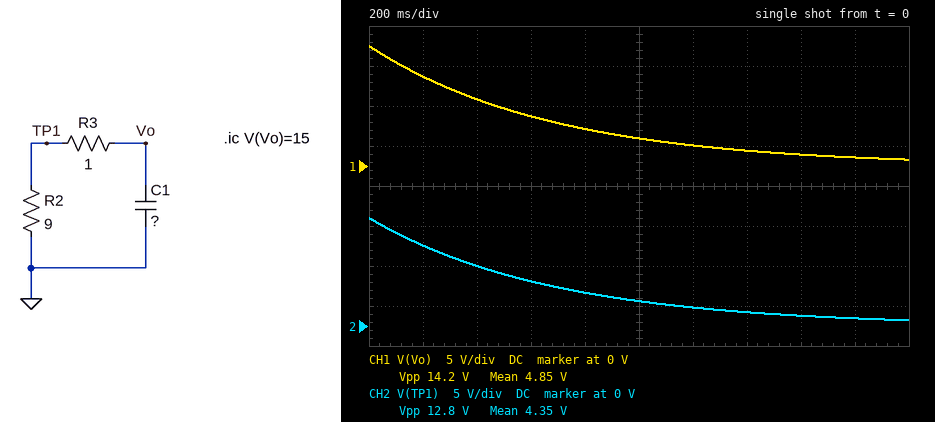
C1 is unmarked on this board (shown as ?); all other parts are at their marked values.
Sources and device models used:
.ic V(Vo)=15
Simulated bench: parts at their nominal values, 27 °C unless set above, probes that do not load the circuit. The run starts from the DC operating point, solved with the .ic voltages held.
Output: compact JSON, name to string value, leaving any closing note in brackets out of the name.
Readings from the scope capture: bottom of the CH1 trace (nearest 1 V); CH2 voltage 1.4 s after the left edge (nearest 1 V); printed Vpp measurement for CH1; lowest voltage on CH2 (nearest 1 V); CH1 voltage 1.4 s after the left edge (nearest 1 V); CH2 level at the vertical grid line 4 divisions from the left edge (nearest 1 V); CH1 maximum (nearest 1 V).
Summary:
{"bottom of the CH1 trace": "1 V", "CH2 voltage 1.4 s after the left edge": "2 V", "printed Vpp measurement for CH1": "14.2 V", "lowest voltage on CH2": "1 V", "CH1 voltage 1.4 s after the left edge": "2 V", "CH2 level at the vertical grid line 4 divisions from the left edge": "4 V", "CH1 maximum": "15 V"}
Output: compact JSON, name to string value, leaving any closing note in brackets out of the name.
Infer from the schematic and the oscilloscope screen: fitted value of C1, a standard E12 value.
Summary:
{"fitted value of C1, a standard E12 value": "68 mF"}
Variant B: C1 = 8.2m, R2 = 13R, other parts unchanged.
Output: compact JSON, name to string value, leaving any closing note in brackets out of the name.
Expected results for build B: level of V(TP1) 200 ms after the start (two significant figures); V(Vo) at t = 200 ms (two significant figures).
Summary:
{"level of V(TP1) 200 ms after the start": "2.4 V", "V(Vo) at t = 200 ms": "2.6 V"}
